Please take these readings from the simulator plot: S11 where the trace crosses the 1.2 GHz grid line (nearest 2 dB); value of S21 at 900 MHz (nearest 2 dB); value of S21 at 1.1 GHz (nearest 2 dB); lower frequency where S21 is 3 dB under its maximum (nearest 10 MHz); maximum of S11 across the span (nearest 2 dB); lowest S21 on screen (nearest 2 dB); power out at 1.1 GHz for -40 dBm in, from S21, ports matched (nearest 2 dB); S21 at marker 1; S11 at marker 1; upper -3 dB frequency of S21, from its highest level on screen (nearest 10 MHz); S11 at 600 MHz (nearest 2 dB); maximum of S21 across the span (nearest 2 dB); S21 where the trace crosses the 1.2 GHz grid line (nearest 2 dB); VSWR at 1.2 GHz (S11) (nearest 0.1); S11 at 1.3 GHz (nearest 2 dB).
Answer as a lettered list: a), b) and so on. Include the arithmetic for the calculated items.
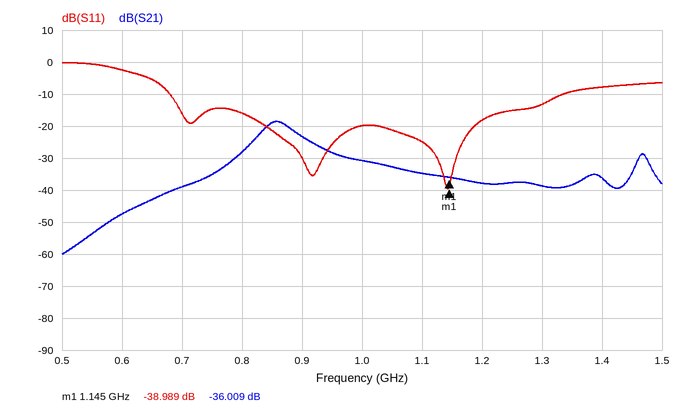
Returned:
a) -18 dB
b) -24 dB
c) -34 dB
d) 830 MHz
e) 0 dB
f) -60 dB
g) -40 dBm + (-34 dB) = -74 dBm
h) -36.009 dB
i) -38.989 dB
j) 890 MHz
k) -2 dB
l) -18 dB
m) -38 dB
n) |Γ| = 10^(-18/20) = 0.1259; VSWR = (1 + 0.1259)/(1 − 0.1259) ≈ 1.3
o) -14 dB
